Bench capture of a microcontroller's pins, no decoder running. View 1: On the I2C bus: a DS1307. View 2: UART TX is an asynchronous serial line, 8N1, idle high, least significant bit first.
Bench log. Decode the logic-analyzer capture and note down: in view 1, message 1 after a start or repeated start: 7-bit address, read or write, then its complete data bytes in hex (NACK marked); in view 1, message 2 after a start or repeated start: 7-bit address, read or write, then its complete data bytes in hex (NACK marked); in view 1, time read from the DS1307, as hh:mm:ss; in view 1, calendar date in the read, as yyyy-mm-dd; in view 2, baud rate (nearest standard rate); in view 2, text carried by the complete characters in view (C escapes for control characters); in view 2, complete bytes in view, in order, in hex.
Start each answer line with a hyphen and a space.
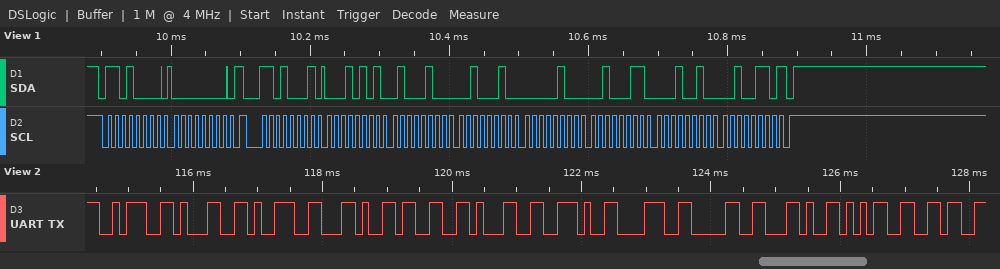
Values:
- 0x68 write: 00
- 0x68 read: 15 44 22 04 23 12 26 NACK
- 22:44:15
- 2026-12-23
- 9600 baud
- ":19,31.80,56"
- 3A 31 39 2C 33 31 2E 38 30 2C 35 36
